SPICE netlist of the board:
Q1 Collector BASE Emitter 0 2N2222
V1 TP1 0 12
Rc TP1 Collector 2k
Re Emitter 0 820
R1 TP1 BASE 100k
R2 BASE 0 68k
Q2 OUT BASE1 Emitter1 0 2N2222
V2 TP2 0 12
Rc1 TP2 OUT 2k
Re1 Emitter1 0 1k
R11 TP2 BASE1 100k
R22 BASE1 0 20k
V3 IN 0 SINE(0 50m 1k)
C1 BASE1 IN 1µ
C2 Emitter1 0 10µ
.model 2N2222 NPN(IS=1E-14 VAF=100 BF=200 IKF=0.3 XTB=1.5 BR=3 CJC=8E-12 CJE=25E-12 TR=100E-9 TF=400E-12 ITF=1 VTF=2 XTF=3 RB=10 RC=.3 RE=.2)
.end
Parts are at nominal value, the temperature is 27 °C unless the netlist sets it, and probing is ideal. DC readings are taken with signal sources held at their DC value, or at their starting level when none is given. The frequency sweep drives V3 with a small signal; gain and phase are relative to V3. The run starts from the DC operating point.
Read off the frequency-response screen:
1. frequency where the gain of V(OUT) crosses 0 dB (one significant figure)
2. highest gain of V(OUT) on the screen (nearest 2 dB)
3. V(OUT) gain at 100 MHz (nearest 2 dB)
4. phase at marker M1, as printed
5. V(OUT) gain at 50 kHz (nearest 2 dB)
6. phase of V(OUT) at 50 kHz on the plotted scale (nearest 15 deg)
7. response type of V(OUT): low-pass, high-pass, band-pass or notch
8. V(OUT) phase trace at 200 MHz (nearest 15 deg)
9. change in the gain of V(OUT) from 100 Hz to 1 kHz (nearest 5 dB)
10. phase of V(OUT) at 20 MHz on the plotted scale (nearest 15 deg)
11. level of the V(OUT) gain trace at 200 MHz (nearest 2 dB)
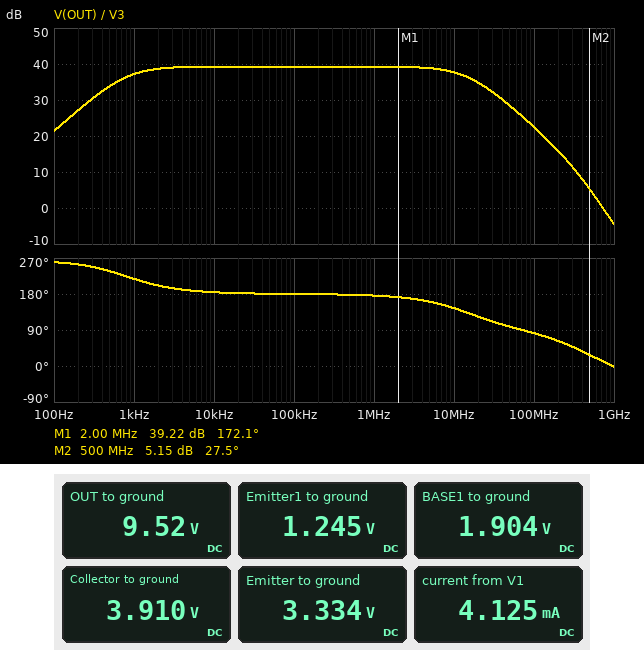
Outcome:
700 MHz
40 dB
22 dB
172.1 deg
40 dB
180 deg
band-pass
60 deg
15 dB
120 deg
16 dB
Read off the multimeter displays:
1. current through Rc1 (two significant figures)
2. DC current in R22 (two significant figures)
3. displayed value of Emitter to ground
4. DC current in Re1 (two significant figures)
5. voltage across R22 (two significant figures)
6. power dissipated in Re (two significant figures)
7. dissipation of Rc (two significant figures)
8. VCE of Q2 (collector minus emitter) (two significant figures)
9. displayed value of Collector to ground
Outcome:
1.2 mA
95 µA
3.334 V
1.2 mA
1.9 V
14 mW
33 mW
8.3 V
3.910 V
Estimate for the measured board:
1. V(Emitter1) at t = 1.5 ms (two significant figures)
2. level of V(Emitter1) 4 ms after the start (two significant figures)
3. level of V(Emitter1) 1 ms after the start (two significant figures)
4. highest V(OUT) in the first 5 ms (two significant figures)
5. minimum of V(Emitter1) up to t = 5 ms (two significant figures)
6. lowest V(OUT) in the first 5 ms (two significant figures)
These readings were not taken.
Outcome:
1.3 V
1.2 V
1.2 V
12 V
1.2 V
5.4 V
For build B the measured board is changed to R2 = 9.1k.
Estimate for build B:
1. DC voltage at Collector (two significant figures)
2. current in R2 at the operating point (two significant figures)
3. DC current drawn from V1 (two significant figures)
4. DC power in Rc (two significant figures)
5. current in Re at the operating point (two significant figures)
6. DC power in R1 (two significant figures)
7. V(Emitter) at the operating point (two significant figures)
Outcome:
11 V
110 µA
540 µA
370 µW
430 µA
1.2 mW
350 mV
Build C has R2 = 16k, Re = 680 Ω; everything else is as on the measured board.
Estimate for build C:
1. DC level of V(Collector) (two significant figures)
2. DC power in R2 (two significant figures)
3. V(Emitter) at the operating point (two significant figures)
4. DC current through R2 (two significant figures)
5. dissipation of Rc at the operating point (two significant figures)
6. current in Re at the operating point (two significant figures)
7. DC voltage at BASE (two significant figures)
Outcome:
9.3 V
150 µW
910 mV
98 µA
3.5 mW
1.3 mA
1.6 V
